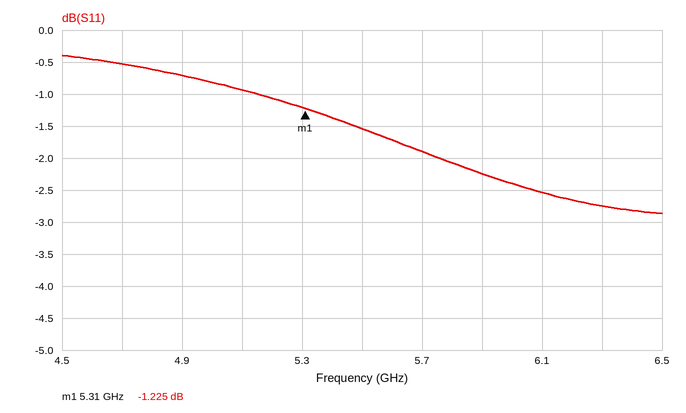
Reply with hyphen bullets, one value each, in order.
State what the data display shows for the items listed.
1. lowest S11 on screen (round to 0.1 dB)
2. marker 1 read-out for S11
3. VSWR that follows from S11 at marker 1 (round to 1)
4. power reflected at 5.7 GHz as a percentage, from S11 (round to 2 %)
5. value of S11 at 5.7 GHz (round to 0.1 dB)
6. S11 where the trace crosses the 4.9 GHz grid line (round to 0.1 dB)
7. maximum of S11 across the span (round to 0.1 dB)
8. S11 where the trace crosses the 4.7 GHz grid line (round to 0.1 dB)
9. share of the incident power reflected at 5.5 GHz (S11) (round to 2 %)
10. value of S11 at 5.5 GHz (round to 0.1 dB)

- -2.9 dB
- -1.225 dB
- 14
- 64 %
- -1.9 dB
- -0.7 dB
- -0.4 dB
- -0.5 dB
- 70 %
- -1.5 dB
